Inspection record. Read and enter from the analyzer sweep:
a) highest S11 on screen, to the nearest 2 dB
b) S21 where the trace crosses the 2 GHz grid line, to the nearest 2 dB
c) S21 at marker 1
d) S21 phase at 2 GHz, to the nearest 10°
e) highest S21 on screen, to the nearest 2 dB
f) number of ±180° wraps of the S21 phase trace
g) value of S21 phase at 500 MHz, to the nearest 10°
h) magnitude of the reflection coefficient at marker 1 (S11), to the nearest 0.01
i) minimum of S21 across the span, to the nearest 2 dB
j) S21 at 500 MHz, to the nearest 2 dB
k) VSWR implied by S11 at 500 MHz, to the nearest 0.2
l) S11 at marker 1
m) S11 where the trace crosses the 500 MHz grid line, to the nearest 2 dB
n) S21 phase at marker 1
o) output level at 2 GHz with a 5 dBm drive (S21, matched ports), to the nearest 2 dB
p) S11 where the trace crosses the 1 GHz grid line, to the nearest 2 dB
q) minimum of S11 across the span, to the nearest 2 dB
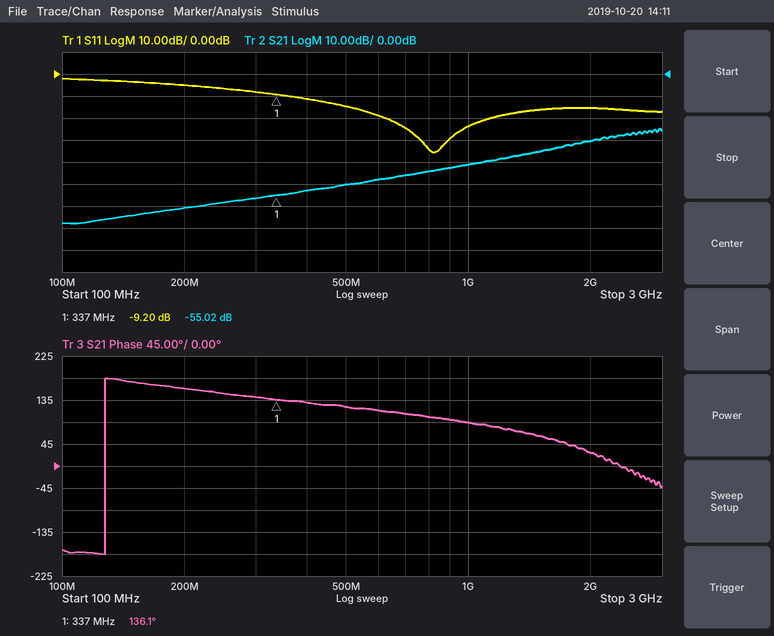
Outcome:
-2 dB
-30 dB
-55.02 dB
30°
-24 dB
1
120°
0.35
-68 dB
-50 dB
1.4
-9.20 dB
-14 dB
136.1°
-26 dBm
-24 dB
-36 dB
